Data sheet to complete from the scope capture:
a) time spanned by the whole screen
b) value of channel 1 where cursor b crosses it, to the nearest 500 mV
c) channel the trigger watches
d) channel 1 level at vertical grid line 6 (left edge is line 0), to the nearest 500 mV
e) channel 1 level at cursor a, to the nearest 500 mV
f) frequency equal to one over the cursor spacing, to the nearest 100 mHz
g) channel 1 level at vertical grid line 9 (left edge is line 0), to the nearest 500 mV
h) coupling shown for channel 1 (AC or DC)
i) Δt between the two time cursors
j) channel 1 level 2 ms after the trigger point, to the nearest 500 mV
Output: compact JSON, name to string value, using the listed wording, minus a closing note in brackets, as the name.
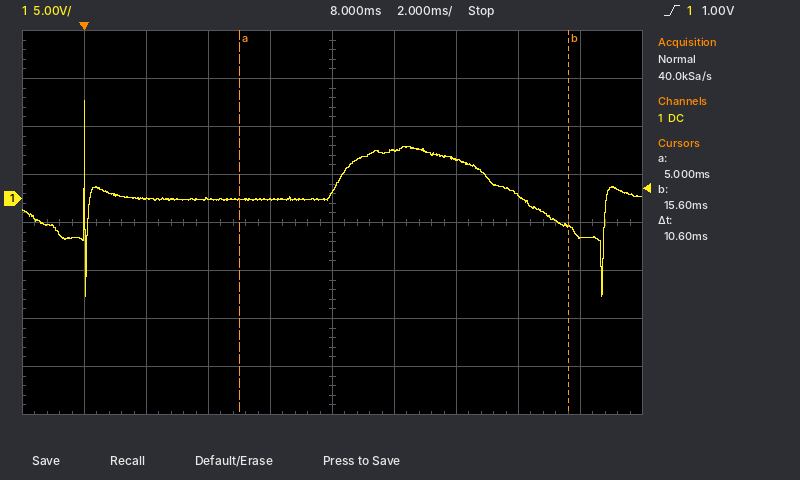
{"time spanned by the whole screen": "20 ms", "value of channel 1 where cursor b crosses it, to the nearest 500 mV": "-3.0 V", "channel the trigger watches": "channel 1", "channel 1 level at vertical grid line 6 (left edge is line 0), to the nearest 500 mV": "5.0 V", "channel 1 level at cursor a, to the nearest 500 mV": "0.0 V", "frequency equal to one over the cursor spacing, to the nearest 100 mHz": "94.3 Hz", "channel 1 level at vertical grid line 9 (left edge is line 0), to the nearest 500 mV": "-4.0 V", "coupling shown for channel 1": "DC", "Δt between the two time cursors": "10.6 ms", "channel 1 level 2 ms after the trigger point, to the nearest 500 mV": "0.0 V"}
